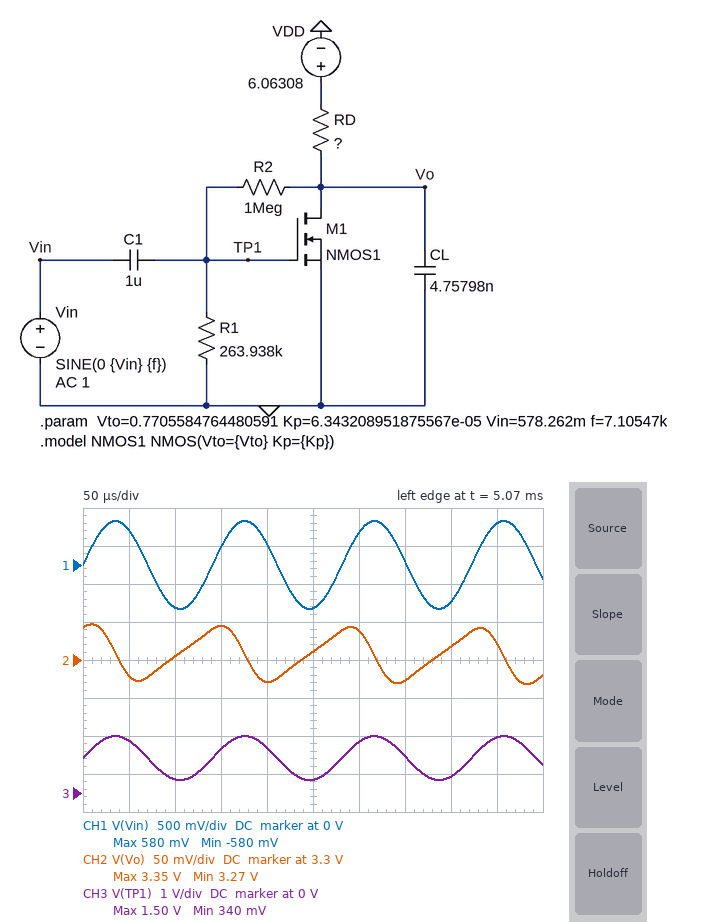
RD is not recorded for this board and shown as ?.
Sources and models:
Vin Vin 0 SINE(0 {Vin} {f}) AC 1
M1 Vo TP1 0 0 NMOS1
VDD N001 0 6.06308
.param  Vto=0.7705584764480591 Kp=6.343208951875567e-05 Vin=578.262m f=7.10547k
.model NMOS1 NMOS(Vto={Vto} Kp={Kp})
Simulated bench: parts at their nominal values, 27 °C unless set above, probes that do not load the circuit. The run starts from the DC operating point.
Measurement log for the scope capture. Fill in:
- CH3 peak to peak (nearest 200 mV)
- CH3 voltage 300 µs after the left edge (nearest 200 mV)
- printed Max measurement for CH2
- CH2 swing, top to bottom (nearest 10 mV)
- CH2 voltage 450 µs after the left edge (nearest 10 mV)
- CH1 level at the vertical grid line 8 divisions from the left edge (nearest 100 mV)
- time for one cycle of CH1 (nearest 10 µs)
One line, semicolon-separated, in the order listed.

1.2 V; 1.4 V; 3.35 V; 80 mV; 3.32 V; -500 mV; 140 µs
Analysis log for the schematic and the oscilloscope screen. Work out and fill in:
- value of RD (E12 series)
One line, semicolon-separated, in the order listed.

390 kΩ
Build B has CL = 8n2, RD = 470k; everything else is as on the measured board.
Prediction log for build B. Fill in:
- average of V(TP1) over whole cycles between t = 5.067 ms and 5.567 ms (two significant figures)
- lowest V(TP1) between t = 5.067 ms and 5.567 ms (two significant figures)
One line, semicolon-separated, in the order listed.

890 mV; 310 mV
